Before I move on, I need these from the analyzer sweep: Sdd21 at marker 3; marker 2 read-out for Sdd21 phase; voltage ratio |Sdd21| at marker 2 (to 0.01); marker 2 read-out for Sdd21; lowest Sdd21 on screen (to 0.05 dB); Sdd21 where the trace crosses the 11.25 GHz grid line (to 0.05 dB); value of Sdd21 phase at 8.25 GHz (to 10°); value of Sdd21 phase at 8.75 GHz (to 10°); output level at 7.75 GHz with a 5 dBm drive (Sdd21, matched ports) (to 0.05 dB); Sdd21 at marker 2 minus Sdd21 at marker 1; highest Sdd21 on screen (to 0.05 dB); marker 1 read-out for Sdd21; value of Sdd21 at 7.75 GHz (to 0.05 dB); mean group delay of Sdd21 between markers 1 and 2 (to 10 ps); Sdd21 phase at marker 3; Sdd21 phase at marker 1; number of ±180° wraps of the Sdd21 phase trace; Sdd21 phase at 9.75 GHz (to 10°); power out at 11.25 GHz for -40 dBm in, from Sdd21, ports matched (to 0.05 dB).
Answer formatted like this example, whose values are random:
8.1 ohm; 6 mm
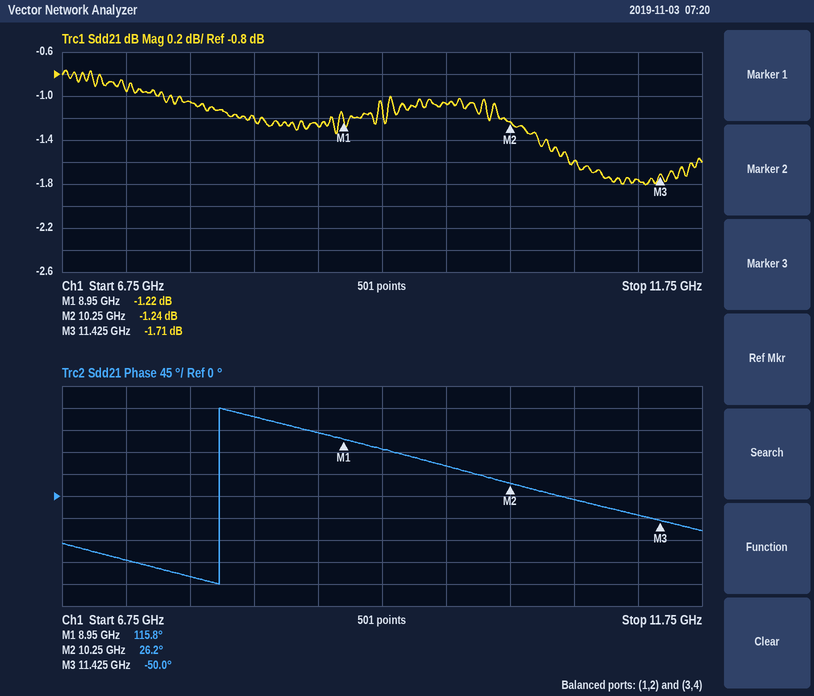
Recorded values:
-1.71 dB; 26.2°; 0.87; -1.24 dB; -1.80 dB; -1.75 dB; 160°; 130°; 3.95 dBm; -0.02 dB; -0.75 dB; -1.22 dB; -1.05 dB; 190 ps; -50.0°; 115.8°; 1; 60°; -41.75 dBm
